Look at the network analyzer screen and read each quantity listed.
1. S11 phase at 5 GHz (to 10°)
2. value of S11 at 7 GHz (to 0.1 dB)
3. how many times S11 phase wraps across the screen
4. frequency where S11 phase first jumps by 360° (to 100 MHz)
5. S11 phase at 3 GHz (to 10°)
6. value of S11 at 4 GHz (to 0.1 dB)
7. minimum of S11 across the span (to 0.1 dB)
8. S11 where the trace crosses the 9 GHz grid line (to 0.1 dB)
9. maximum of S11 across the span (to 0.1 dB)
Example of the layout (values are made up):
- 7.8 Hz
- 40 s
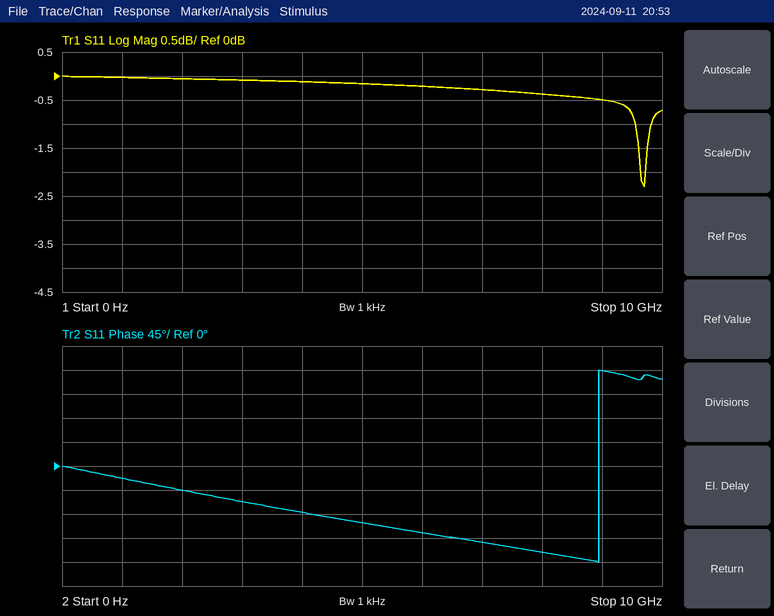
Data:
- -110°
- -0.3 dB
- 1
- 8.9 GHz
- -70°
- -0.1 dB
- -2.3 dB
- -0.5 dB
- 0.0 dB
